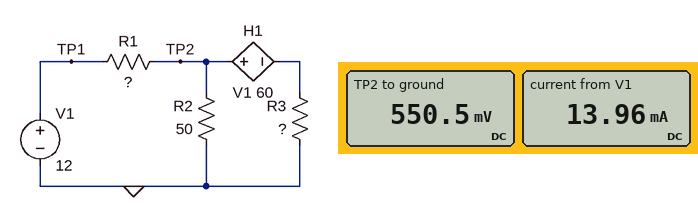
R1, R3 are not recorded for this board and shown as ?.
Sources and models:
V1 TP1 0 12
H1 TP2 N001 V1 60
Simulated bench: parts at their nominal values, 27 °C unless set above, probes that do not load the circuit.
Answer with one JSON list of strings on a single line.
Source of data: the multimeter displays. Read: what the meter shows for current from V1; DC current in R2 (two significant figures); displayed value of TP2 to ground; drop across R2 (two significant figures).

["13.96 mA", "11 mA", "550.5 mV", "550 mV"]
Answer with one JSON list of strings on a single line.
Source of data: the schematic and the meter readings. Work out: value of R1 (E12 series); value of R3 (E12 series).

["820 Ω", "470 Ω"]
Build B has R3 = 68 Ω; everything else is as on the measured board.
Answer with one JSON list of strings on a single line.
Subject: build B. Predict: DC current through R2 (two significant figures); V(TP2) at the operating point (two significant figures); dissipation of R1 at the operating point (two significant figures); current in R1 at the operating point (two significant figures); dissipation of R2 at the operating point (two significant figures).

["990 µA", "49 mV", "170 mW", "15 mA", "49 µW"]
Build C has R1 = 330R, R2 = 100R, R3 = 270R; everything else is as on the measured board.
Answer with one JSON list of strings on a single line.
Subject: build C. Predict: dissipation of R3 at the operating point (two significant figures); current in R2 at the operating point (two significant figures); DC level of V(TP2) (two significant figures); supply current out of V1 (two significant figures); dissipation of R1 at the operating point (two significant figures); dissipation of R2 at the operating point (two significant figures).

["49 mW", "18 mA", "1.8 V", "31 mA", "320 mW", "31 mW"]
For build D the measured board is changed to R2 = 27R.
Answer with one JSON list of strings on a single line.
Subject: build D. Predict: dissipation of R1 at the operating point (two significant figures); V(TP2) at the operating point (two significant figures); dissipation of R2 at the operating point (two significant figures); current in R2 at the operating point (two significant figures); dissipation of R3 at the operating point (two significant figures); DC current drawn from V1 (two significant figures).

["170 mW", "320 mV", "3.7 mW", "12 mA", "2.9 mW", "14 mA"]
